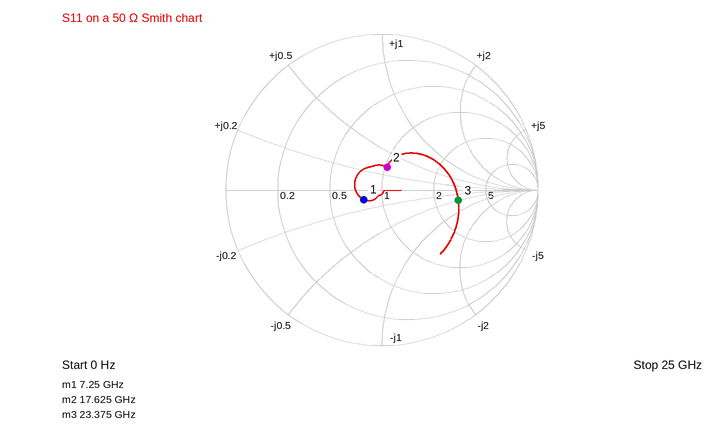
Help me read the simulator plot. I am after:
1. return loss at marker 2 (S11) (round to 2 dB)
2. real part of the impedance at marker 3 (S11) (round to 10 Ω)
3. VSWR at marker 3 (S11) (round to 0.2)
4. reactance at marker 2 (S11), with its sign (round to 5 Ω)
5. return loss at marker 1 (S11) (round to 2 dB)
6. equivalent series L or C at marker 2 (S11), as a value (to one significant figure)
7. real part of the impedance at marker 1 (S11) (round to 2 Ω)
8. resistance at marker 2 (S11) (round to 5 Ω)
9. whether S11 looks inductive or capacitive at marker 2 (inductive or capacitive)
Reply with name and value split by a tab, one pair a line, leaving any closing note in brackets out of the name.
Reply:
return loss at marker 2 (S11)	16 dB
real part of the impedance at marker 3 (S11)	140 Ω
VSWR at marker 3 (S11)	3.0
reactance at marker 2 (S11), with its sign	+15 Ω
return loss at marker 1 (S11)	18 dB
equivalent series L or C at marker 2 (S11), as a value	100 pH
real part of the impedance at marker 1 (S11)	40 Ω
resistance at marker 2 (S11)	50 Ω
whether S11 looks inductive or capacitive at marker 2	inductive
